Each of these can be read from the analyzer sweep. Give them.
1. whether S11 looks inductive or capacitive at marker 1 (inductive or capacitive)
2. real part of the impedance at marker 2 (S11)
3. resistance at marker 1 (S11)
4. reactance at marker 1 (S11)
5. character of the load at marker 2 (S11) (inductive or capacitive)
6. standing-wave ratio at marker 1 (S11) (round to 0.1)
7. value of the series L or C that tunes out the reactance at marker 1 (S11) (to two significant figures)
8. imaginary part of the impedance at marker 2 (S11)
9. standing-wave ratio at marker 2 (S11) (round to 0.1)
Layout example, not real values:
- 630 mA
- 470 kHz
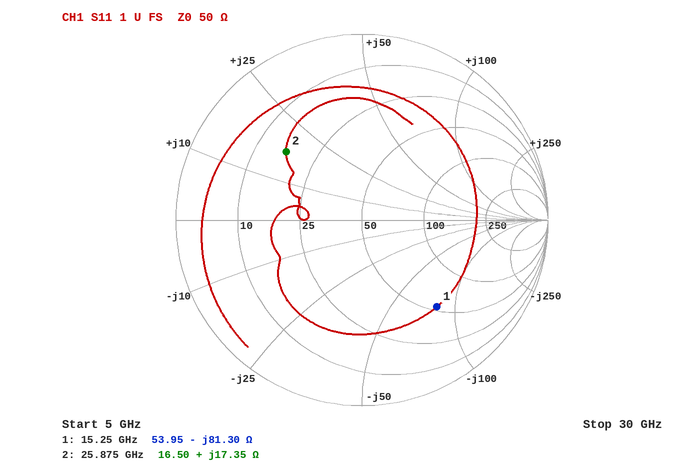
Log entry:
- capacitive
- 16.50 Ω
- 53.95 Ω
- -81.30 Ω
- inductive
- 4.2
- 850 pH
- +17.35 Ω
- 3.4
